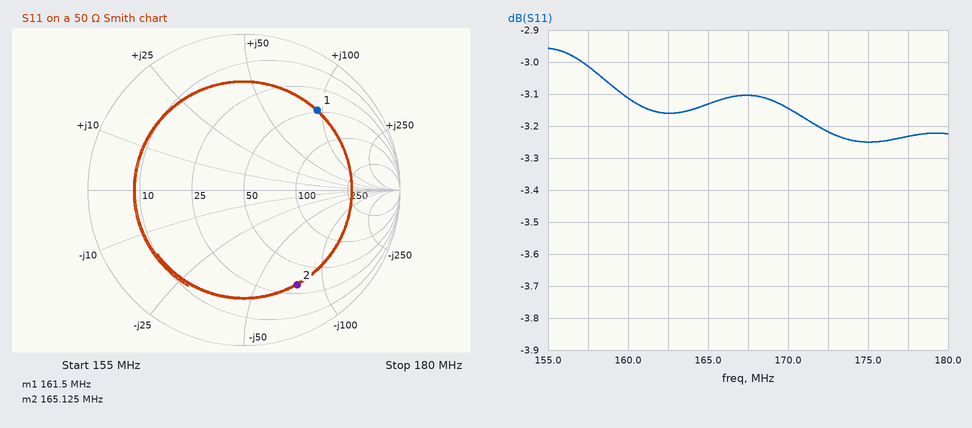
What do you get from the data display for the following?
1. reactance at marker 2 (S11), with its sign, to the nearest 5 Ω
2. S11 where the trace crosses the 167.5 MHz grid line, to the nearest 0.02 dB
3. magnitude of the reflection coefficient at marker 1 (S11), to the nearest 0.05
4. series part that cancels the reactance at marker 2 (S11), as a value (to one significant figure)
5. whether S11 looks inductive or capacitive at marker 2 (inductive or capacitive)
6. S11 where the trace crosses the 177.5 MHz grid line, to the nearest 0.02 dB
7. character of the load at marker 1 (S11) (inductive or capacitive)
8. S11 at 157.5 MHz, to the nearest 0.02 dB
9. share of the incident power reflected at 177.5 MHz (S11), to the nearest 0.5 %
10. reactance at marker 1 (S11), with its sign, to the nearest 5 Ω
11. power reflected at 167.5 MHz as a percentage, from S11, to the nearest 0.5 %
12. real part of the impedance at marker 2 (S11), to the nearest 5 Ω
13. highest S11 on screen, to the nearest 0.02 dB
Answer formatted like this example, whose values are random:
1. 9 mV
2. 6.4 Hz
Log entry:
1. -75 Ω
2. -3.10 dB
3. 0.70
4. 70 nH
5. capacitive
6. -3.24 dB
7. inductive
8. -3.02 dB
9. 47.5 %
10. +95 Ω
11. 49.0 %
12. 30 Ω
13. -2.96 dB
